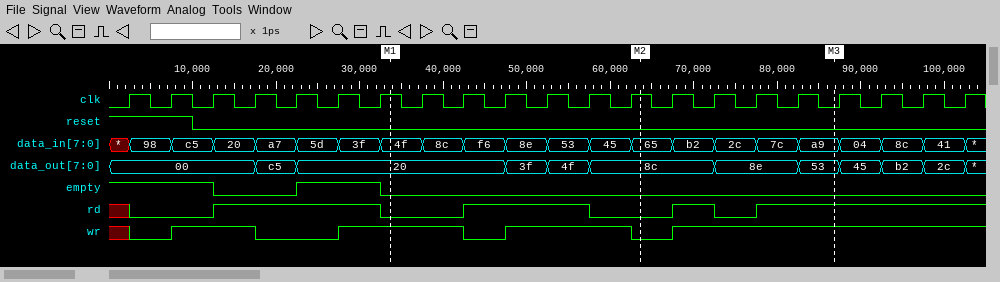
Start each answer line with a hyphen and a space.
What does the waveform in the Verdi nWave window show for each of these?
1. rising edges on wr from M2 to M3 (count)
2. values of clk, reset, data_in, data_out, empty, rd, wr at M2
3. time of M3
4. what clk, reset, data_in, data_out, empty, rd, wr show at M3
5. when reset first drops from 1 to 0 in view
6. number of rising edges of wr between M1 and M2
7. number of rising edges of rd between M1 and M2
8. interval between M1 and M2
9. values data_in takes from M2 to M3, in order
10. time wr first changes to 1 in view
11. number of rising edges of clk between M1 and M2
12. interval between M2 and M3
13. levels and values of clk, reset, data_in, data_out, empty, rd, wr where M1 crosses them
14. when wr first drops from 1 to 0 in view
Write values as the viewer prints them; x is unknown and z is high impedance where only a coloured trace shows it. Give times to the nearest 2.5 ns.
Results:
- 1
- clk=1, reset=0, data_in=65, data_out=8c, empty=0, rd=0, wr=0
- 87.5 ns
- clk=0, reset=0, data_in=a9, data_out=53, empty=0, rd=1, wr=1
- 10 ns
- 1
- 1
- 30 ns
- 65, b2, 2c, 7c, a9
- 7.5 ns
- 6
- 22.5 ns
- clk=1, reset=0, data_in=4f, data_out=20, empty=0, rd=0, wr=1
- 17.5 ns
